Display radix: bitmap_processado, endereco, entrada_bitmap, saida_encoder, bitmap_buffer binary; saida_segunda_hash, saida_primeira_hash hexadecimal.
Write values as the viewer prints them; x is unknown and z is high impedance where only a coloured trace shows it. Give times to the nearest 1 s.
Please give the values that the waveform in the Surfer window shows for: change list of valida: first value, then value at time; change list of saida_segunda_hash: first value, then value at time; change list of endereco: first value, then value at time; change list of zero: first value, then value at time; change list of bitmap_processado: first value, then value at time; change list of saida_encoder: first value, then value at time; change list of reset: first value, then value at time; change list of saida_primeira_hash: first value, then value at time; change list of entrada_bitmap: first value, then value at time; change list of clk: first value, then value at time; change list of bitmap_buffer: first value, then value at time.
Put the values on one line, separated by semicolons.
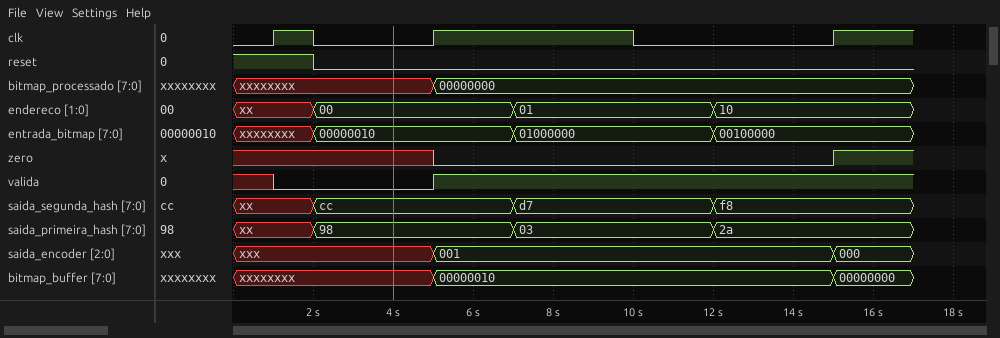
x, 0 at 1 s, 1 at 5 s; xx, cc at 2 s, d7 at 7 s, f8 at 12 s; xx, 00 at 2 s, 01 at 7 s, 10 at 12 s; x, 0 at 5 s, 1 at 15 s; xxxxxxxx, 00000000 at 5 s; xxx, 001 at 5 s, 000 at 15 s; 1, 0 at 2 s; xx, 98 at 2 s, 03 at 7 s, 2a at 12 s; xxxxxxxx, 00000010 at 2 s, 01000000 at 7 s, 00100000 at 12 s; 0, 1 at 1 s, 0 at 2 s, 1 at 5 s, 0 at 10 s, 1 at 15 s; xxxxxxxx, 00000010 at 5 s, 00000000 at 15 s
